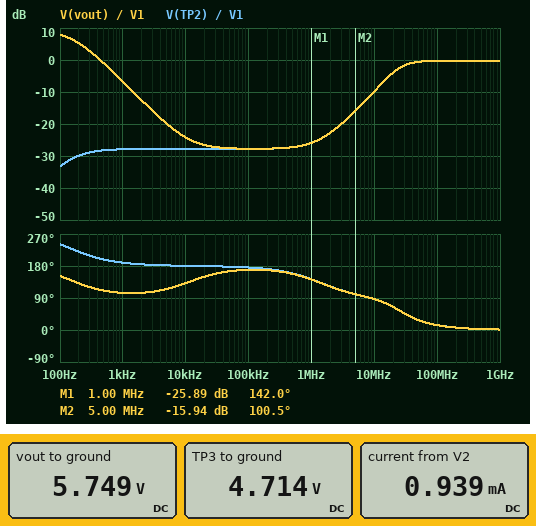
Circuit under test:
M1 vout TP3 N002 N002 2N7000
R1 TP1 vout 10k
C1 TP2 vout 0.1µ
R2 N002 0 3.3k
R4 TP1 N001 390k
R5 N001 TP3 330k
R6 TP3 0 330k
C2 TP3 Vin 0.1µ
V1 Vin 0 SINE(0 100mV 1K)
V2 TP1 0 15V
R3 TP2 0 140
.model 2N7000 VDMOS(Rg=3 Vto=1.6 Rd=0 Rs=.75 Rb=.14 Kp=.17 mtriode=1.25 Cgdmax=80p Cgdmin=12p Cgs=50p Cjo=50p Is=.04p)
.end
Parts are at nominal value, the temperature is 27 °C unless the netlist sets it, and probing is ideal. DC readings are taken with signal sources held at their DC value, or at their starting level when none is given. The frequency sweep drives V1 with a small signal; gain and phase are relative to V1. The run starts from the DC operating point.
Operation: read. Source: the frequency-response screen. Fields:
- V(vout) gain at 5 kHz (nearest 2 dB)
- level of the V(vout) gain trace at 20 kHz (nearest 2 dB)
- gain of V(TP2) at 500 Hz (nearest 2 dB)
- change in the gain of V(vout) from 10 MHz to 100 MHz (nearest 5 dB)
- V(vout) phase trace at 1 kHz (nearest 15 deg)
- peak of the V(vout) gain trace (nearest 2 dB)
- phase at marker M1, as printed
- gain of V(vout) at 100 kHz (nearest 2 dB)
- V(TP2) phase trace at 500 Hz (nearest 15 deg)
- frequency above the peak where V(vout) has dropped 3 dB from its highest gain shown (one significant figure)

-20 dB
-26 dB
-28 dB
10 dB
105 deg
8 dB
142.0 deg
-28 dB
195 deg
200 Hz
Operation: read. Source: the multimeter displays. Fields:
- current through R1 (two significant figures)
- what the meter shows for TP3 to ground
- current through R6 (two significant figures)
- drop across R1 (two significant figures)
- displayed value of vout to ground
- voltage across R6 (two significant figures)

930 µA
4.714 V
14 µA
9.3 V
5.749 V
4.7 V
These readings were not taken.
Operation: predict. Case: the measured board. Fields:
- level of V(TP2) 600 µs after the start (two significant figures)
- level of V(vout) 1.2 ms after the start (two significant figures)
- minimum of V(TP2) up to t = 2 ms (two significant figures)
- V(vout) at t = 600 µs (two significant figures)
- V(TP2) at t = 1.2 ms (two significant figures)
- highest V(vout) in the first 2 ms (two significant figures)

3.2 mV
5.7 V
-3.8 mV
5.7 V
-3.8 mV
5.8 V
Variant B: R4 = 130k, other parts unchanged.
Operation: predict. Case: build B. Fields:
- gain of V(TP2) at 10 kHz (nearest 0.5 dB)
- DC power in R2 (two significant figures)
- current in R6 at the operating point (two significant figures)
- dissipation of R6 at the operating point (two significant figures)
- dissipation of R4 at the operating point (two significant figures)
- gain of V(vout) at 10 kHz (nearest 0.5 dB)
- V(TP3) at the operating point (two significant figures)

-59.0 dB
4.2 mW
19 µA
120 µW
47 µW
-55.5 dB
6.3 V
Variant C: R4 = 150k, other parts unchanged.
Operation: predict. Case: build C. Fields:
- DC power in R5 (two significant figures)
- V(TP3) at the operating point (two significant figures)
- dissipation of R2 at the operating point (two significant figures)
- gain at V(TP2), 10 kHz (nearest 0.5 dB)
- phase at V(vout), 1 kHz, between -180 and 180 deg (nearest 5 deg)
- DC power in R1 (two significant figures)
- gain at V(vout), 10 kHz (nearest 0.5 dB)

110 µW
6.1 V
4.2 mW
-59.0 dB
110 deg
13 mW
-55.5 dB
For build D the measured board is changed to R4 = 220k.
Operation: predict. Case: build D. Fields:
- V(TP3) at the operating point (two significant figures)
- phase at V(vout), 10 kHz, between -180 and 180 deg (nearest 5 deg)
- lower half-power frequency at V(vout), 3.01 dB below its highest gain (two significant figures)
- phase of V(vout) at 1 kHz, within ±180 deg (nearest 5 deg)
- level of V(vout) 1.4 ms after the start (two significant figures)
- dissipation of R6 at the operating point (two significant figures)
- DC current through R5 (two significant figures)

5.6 V
110 deg
9.5 MHz
125 deg
3.7 V
96 µW
17 µA
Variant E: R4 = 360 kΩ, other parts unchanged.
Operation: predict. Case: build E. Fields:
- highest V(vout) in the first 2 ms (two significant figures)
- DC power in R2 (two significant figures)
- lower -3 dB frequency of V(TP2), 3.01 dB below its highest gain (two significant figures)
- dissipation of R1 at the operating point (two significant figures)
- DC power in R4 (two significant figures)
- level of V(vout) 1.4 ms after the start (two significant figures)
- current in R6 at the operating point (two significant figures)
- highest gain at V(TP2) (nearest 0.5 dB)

5.4 V
3.1 mW
19 MHz
9.3 mW
78 µW
5.3 V
15 µA
0 dB
